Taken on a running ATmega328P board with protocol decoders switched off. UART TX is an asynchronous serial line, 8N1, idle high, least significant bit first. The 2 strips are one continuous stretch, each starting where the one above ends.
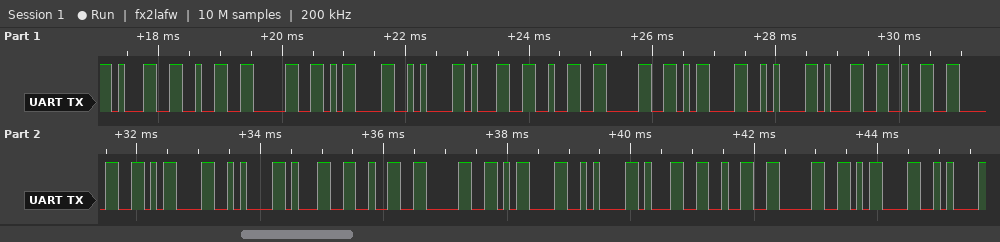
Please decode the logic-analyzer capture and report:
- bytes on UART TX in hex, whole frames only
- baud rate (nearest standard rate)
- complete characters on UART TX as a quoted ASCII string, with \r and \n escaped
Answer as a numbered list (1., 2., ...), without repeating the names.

1. 31 32 30 0D 0A 31 32 30 0D 0A 31 32 30 0D 0A 31 32 30 0D 0A 31 32 30 0D 0A
2. 9600 baud
3. "120\r\n120\r\n120\r\n120\r\n120\r\n"
